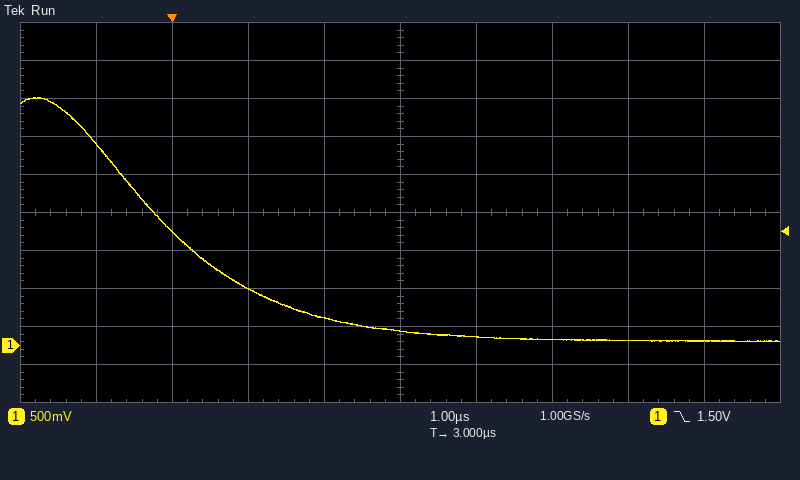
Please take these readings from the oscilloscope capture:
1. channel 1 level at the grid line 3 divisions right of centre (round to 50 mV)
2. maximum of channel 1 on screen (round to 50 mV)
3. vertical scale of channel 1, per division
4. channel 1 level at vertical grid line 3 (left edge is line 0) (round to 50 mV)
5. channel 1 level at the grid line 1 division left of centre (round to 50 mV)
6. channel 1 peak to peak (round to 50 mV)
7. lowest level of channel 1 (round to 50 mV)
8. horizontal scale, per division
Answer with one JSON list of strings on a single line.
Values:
["50 mV", "3.25 V", "500 mV", "750 mV", "350 mV", "3.20 V", "50 mV", "1 µs"]
